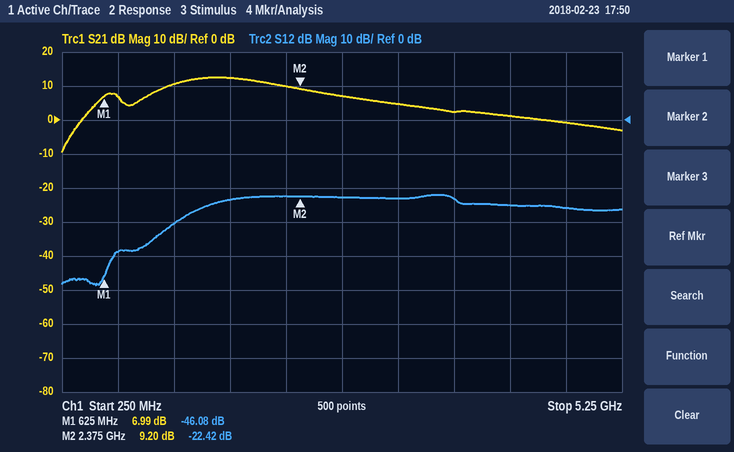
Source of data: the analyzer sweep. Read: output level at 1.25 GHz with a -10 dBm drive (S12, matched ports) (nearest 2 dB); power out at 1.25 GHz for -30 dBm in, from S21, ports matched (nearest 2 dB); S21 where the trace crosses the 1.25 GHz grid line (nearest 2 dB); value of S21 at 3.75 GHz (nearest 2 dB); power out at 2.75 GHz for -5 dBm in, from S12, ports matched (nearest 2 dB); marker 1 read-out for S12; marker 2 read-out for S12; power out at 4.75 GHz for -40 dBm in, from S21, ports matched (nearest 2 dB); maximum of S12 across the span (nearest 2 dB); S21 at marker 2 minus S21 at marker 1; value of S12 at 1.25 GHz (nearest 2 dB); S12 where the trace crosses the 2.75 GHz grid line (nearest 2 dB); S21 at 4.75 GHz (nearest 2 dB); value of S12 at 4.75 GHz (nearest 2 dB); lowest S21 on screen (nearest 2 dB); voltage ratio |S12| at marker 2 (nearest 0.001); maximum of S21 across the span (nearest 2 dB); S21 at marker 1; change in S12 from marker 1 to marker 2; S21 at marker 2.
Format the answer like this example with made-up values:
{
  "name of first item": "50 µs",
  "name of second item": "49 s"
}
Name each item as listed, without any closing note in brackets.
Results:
{
  "output level at 1.25 GHz with a -10 dBm drive (S12, matched ports)": "-40 dBm",
  "power out at 1.25 GHz for -30 dBm in, from S21, ports matched": "-20 dBm",
  "S21 where the trace crosses the 1.25 GHz grid line": "10 dB",
  "value of S21 at 3.75 GHz": "2 dB",
  "power out at 2.75 GHz for -5 dBm in, from S12, ports matched": "-28 dBm",
  "marker 1 read-out for S12": "-46.08 dB",
  "marker 2 read-out for S12": "-22.42 dB",
  "power out at 4.75 GHz for -40 dBm in, from S21, ports matched": "-40 dBm",
  "maximum of S12 across the span": "-22 dB",
  "S21 at marker 2 minus S21 at marker 1": "2.21 dB",
  "value of S12 at 1.25 GHz": "-30 dB",
  "S12 where the trace crosses the 2.75 GHz grid line": "-22 dB",
  "S21 at 4.75 GHz": "0 dB",
  "value of S12 at 4.75 GHz": "-26 dB",
  "lowest S21 on screen": "-10 dB",
  "voltage ratio |S12| at marker 2": "0.076",
  "maximum of S21 across the span": "12 dB",
  "S21 at marker 1": "6.99 dB",
  "change in S12 from marker 1 to marker 2": "23.66 dB",
  "S21 at marker 2": "9.20 dB"
}
